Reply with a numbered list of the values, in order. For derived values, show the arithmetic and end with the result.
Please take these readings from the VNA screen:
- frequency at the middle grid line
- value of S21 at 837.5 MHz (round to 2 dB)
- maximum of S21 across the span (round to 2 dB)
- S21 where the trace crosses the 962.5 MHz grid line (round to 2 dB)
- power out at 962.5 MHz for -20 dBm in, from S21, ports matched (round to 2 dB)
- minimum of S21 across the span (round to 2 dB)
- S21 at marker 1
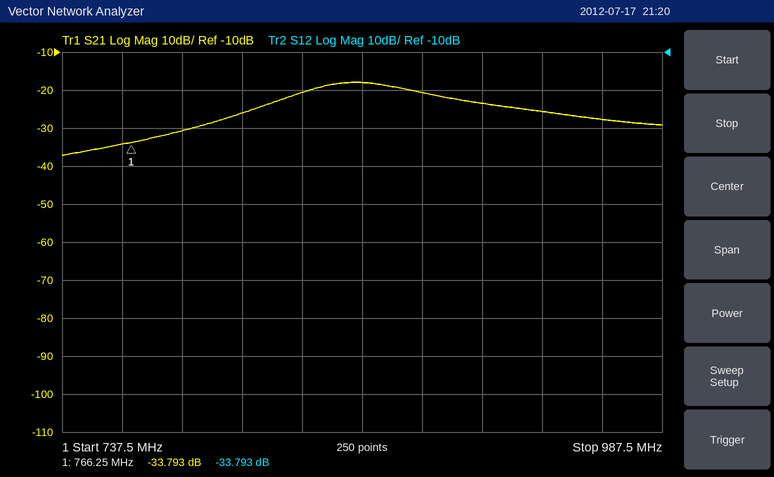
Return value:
1. 862.5 MHz
2. -20 dB
3. -18 dB
4. -28 dB
5. -20 dBm + (-28 dB) = -48 dBm
6. -38 dB
7. -33.793 dB
